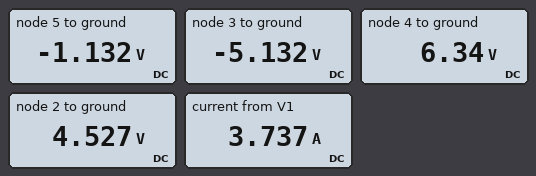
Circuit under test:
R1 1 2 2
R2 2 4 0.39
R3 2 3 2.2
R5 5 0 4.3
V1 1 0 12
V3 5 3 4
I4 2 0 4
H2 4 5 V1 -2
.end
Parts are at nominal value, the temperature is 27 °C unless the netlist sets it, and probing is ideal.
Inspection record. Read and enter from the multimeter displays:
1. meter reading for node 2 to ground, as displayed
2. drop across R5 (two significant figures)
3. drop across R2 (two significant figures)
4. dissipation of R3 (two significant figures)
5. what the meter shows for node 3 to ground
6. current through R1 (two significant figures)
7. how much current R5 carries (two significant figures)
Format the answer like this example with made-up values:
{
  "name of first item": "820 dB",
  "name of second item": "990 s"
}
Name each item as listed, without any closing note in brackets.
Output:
{
  "meter reading for node 2 to ground, as displayed": "4.527 V",
  "drop across R5": "1.1 V",
  "drop across R2": "1.8 V",
  "dissipation of R3": "42 W",
  "what the meter shows for node 3 to ground": "-5.132 V",
  "current through R1": "3.7 A",
  "how much current R5 carries": "260 mA"
}
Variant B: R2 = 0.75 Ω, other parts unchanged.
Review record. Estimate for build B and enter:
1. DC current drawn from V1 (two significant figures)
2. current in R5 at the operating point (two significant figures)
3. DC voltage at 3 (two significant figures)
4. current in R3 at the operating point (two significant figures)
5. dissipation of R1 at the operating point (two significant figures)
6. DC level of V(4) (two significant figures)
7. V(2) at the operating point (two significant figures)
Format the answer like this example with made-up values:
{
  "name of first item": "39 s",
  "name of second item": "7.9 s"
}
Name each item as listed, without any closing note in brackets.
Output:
{
  "DC current drawn from V1": "3.9 A",
  "current in R5 at the operating point": "110 mA",
  "DC voltage at 3": "-4.5 V",
  "current in R3 at the operating point": "4.0 A",
  "dissipation of R1 at the operating point": "30 W",
  "DC level of V(4)": "7.3 V",
  "V(2) at the operating point": "4.2 V"
}
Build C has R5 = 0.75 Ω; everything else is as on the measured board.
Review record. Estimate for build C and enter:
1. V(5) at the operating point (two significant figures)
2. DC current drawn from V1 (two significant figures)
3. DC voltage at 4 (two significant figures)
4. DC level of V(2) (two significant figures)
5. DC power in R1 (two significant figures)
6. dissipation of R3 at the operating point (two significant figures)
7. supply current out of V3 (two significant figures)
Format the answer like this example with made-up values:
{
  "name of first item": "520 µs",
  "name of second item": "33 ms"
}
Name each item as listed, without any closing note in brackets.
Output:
{
  "V(5) at the operating point": "-340 mV",
  "DC current drawn from V1": "3.5 A",
  "DC voltage at 4": "6.7 V",
  "DC level of V(2)": "4.9 V",
  "DC power in R1": "25 W",
  "dissipation of R3 at the operating point": "39 W",
  "supply current out of V3": "4.2 A"
}
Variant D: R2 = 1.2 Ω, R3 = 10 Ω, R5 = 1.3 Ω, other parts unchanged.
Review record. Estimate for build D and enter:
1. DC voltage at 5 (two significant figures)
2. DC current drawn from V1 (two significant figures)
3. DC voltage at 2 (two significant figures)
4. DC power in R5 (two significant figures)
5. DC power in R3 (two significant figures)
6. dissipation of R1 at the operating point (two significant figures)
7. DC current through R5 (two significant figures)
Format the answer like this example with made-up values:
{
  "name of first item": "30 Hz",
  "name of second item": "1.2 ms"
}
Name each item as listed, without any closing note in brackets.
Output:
{
  "DC voltage at 5": "-570 mV",
  "DC current drawn from V1": "3.6 A",
  "DC voltage at 2": "4.9 V",
  "DC power in R5": "250 mW",
  "DC power in R3": "8.9 W",
  "dissipation of R1 at the operating point": "25 W",
  "DC current through R5": "440 mA"
}
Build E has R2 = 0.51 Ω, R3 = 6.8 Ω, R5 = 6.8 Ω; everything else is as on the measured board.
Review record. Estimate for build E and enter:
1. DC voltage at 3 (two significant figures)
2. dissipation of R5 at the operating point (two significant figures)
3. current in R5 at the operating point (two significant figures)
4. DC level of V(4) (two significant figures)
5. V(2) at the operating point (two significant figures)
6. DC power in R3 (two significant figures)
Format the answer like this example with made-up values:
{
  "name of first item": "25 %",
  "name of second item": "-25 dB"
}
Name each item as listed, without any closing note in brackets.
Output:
{
  "DC voltage at 3": "-5.9 V",
  "dissipation of R5 at the operating point": "550 mW",
  "current in R5 at the operating point": "280 mA",
  "DC level of V(4)": "5.5 V",
  "V(2) at the operating point": "4.6 V",
  "DC power in R3": "16 W"
}
